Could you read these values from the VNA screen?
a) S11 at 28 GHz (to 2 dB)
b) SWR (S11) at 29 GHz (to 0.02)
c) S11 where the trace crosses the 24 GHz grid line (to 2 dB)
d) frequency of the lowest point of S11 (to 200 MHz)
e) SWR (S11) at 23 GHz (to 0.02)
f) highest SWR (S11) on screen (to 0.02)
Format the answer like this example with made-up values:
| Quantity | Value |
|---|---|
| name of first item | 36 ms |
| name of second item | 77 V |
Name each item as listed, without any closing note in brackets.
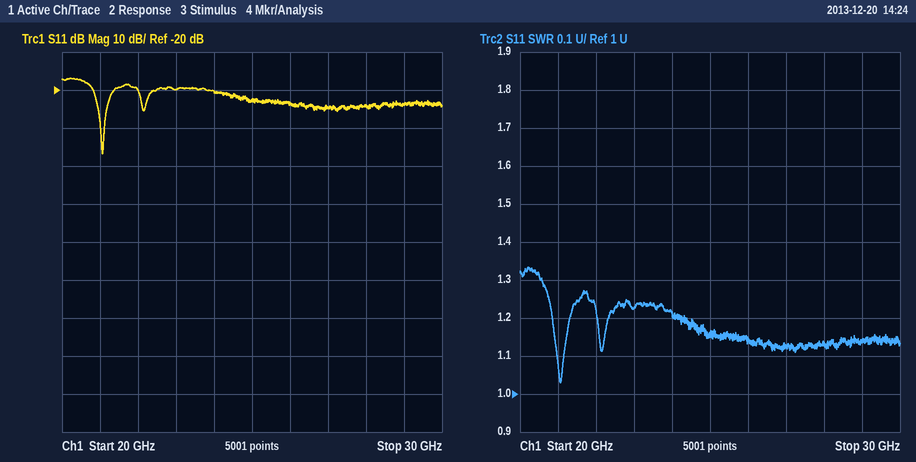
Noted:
| Quantity | Value |
|---|---|
| S11 at 28 GHz | -24 dB |
| SWR (S11) at 29 GHz | 1.14 |
| S11 where the trace crosses the 24 GHz grid line | -20 dB |
| frequency of the lowest point of S11 | 21.0 GHz |
| SWR (S11) at 23 GHz | 1.22 |
| highest SWR (S11) on screen | 1.34 |
